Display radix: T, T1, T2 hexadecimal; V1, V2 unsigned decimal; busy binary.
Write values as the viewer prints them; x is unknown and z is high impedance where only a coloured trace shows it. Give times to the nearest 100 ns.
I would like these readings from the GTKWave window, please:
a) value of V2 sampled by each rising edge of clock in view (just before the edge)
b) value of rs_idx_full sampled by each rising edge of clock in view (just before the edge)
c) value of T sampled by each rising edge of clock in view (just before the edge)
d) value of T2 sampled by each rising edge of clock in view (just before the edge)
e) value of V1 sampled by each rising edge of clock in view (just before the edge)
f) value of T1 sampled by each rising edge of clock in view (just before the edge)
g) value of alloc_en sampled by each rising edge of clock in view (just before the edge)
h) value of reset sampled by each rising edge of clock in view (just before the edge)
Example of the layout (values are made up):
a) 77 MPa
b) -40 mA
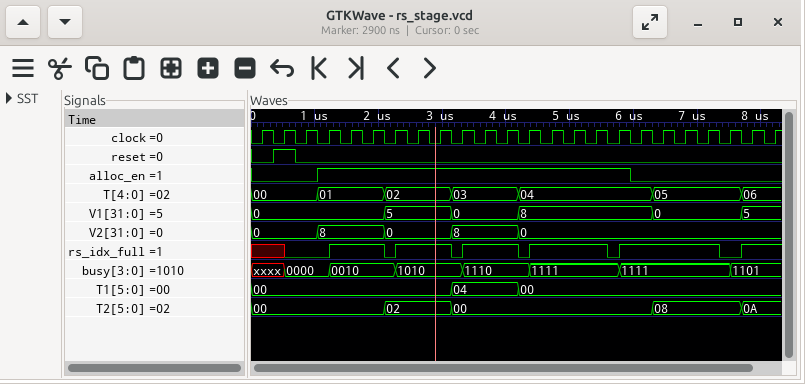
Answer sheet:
a) 0, 0, 0, 8, 8, 8, 0, 0, 0, 8, 8, 8, 0, 0, 0, 0, 0, 0, 0, 0, 0, 0, 0, 0
b) x x 0 0 1 1 0 1 1 0 1 1 0 1 1 1 0 1 1 1 1 0 1 1
c) 00, 00, 00, 01, 01, 01, 02, 02, 02, 03, 03, 03, 04, 04, 04, 04, 04, 04, 05, 05, 05, 05, 06, 06
d) 00, 00, 00, 00, 00, 00, 02, 02, 02, 00, 00, 00, 00, 00, 00, 00, 00, 00, 08, 08, 08, 08, 0A, 0A
e) 0, 0, 0, 0, 0, 0, 5, 5, 5, 0, 0, 0, 8, 8, 8, 8, 8, 8, 0, 0, 0, 0, 5, 5
f) 00, 00, 00, 00, 00, 00, 00, 00, 00, 04, 04, 04, 00, 00, 00, 00, 00, 00, 00, 00, 00, 00, 00, 00
g) 0 0 0 1 1 1 1 1 1 1 1 1 1 1 1 1 1 0 0 0 0 0 0 0
h) 0 1 0 0 0 0 0 0 0 0 0 0 0 0 0 0 0 0 0 0 0 0 0 0
